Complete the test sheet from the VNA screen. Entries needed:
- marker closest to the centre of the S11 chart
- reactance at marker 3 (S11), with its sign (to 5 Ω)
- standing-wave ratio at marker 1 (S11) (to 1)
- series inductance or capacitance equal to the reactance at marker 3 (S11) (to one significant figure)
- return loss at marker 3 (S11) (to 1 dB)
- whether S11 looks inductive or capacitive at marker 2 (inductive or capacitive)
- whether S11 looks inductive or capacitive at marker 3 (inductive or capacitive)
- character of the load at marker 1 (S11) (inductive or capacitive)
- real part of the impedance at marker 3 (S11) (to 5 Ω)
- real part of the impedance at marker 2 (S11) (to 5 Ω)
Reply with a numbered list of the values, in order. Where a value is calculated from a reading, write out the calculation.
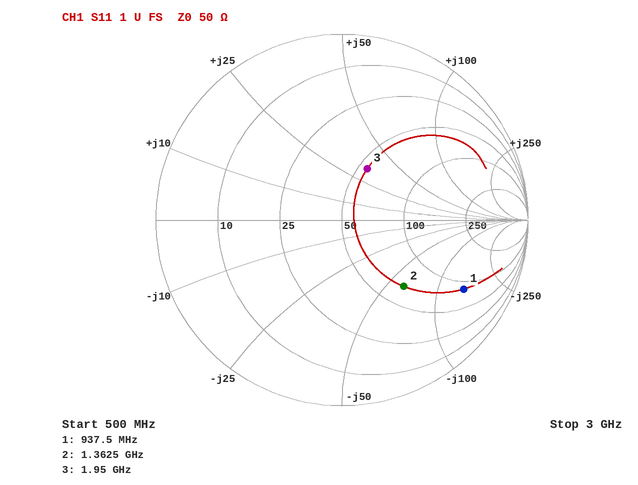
1. marker 3
2. +35 Ω
3. 7
4. L = 35 Ω/(2π × 1.95 GHz) ≈ 3 nH
5. 10 dB
6. capacitive
7. inductive
8. capacitive
9. 55 Ω
10. 65 Ω
